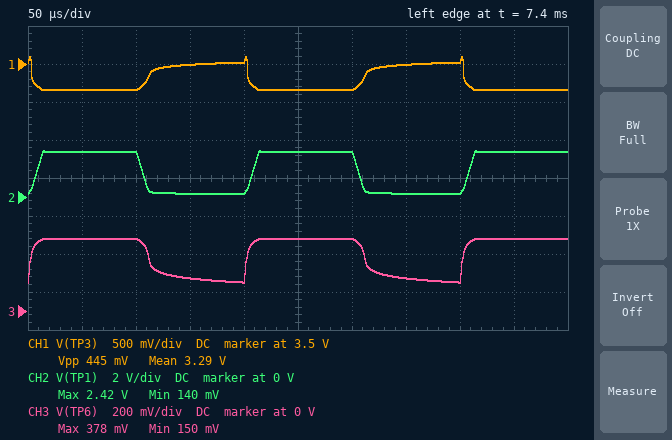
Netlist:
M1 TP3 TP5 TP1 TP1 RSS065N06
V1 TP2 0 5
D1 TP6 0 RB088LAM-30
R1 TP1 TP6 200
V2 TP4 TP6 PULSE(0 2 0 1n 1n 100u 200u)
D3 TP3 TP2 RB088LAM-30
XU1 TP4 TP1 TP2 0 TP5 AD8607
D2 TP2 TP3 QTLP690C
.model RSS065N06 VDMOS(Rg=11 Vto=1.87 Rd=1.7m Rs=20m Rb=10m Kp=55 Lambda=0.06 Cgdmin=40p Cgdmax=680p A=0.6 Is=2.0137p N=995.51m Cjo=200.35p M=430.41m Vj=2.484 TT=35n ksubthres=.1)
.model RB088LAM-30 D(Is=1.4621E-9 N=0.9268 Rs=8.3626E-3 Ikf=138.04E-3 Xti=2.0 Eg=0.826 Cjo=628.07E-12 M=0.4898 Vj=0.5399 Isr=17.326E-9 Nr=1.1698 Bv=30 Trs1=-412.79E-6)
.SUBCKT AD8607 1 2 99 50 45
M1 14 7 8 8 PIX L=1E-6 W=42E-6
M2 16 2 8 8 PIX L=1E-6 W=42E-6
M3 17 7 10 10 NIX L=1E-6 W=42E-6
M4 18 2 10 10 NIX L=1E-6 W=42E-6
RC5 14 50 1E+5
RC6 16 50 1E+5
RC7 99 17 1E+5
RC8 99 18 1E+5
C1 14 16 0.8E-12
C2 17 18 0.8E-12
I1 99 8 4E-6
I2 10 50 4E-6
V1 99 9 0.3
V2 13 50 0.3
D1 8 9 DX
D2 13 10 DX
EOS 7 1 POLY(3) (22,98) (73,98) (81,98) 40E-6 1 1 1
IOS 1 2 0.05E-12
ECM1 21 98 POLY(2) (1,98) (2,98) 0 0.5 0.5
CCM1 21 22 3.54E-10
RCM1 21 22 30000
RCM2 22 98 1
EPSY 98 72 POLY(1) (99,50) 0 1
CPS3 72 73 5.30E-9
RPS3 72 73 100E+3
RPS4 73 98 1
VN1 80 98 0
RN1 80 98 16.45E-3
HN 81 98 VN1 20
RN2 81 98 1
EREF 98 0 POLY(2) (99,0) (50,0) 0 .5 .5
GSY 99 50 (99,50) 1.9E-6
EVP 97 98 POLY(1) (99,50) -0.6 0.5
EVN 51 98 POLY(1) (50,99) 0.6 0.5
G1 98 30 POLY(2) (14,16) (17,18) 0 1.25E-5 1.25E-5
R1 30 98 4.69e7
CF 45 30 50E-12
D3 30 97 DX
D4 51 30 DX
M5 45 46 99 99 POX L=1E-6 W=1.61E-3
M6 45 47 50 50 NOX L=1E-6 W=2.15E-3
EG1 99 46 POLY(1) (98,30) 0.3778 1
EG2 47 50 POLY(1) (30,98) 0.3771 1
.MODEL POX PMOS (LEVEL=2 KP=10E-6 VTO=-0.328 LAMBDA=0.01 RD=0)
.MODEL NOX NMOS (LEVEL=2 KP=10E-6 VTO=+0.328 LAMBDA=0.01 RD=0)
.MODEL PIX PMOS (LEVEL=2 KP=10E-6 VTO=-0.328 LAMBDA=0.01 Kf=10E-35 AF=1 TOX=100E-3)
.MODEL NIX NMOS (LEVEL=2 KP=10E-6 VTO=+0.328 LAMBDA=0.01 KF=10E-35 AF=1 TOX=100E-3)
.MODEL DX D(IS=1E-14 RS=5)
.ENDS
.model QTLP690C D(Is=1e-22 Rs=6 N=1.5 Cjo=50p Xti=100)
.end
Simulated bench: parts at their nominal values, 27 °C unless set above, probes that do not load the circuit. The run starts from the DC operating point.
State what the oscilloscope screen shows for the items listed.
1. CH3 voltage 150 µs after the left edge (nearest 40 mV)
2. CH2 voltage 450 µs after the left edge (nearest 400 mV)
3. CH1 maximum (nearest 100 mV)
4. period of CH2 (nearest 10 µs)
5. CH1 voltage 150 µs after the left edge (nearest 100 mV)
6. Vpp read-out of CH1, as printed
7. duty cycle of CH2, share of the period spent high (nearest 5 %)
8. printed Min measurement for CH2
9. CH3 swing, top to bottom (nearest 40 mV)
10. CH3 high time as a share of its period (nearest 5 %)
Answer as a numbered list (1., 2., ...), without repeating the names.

1. 160 mV
2. 2.4 V
3. 3.6 V
4. 200 µs
5. 3.5 V
6. 445 mV
7. 50 %
8. 140 mV
9. 240 mV
10. 55 %
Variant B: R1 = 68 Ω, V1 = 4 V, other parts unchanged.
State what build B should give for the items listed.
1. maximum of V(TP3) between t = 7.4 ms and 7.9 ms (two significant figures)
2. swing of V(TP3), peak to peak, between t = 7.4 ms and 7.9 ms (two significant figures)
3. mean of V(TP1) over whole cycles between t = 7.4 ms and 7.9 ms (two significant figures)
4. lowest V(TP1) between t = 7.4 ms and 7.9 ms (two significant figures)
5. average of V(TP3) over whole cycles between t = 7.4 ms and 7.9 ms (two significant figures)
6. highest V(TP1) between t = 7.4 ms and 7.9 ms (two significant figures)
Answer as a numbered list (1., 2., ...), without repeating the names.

1. 2.5 V
2. 510 mV
3. 1.2 V
4. 180 mV
5. 2.2 V
6. 2.0 V
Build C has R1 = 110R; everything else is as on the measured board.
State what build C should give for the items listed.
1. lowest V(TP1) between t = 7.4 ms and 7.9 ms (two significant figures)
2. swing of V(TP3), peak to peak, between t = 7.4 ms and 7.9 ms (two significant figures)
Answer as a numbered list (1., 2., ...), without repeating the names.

1. 160 mV
2. 480 mV
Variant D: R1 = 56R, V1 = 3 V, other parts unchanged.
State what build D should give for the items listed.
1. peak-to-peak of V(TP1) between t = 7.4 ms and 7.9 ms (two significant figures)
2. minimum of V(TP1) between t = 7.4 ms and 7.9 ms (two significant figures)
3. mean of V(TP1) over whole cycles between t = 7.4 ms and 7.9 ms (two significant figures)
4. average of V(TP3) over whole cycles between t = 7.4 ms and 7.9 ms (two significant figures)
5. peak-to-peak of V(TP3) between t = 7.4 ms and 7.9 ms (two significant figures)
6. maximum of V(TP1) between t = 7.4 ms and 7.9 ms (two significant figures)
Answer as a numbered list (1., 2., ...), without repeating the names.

1. 940 mV
2. 180 mV
3. 690 mV
4. 1.3 V
5. 430 mV
6. 1.1 V
